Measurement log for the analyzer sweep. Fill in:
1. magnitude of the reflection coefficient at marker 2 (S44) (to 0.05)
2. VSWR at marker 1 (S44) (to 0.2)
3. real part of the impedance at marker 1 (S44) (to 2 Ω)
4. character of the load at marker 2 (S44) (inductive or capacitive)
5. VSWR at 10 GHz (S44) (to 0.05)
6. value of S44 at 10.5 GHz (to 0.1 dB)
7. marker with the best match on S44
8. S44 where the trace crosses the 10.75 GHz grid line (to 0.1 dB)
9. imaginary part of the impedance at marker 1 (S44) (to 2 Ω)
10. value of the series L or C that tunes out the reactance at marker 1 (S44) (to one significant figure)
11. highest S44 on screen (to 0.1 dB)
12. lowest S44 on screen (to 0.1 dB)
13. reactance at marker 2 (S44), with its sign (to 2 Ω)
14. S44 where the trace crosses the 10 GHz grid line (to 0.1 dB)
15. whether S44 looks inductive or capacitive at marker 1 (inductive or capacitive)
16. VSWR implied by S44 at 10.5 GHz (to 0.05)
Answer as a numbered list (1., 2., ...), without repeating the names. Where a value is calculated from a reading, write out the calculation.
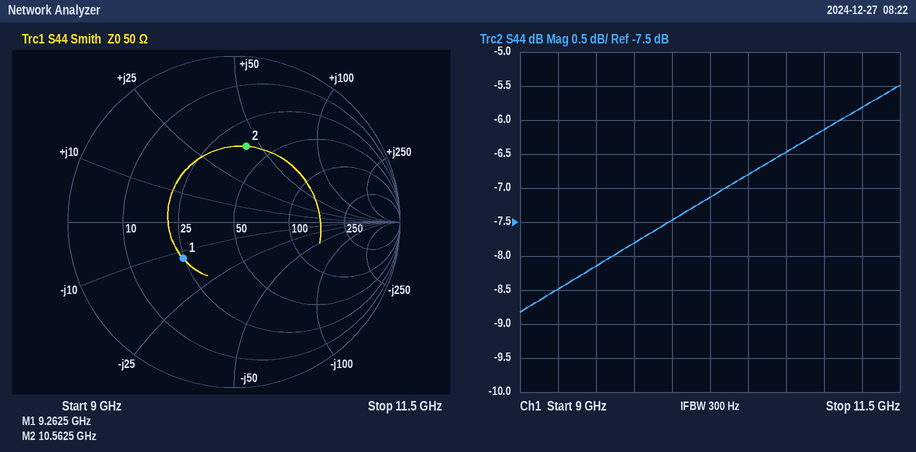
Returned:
1. 0.45
2. 2.2
3. 24 Ω
4. inductive
5. |Γ| = 10^(-7.5/20) = 0.4217; VSWR = (1 + 0.4217)/(1 − 0.4217) ≈ 2.46, so 2.45 to the nearest 0.05
6. -6.8 dB
7. marker 1
8. -6.5 dB
9. -12 Ω
10. L = 12 Ω/(2π × 9.2625 GHz) ≈ 206 pH, so 200 pH to one significant figure
11. -5.5 dB
12. -8.8 dB
13. +42 Ω
14. -7.5 dB
15. capacitive
16. |Γ| = 10^(-6.8/20) = 0.4571; VSWR = (1 + 0.4571)/(1 − 0.4571) ≈ 2.68, so 2.70 to the nearest 0.05
